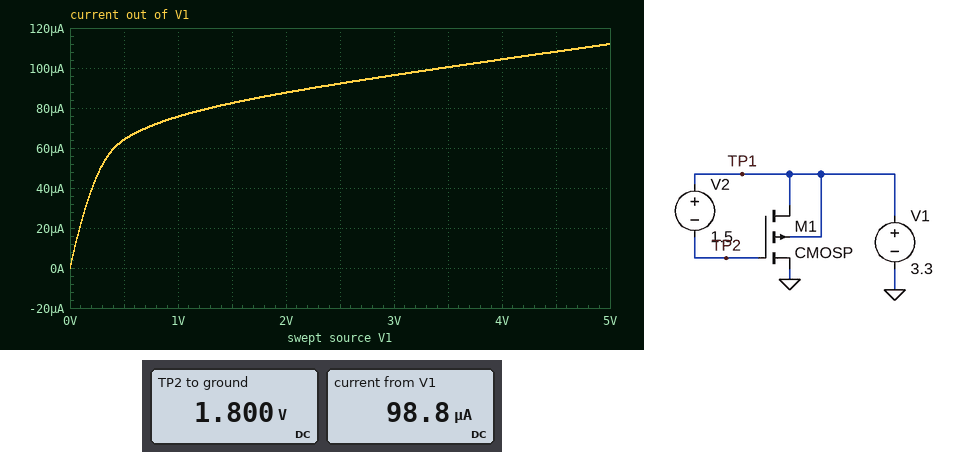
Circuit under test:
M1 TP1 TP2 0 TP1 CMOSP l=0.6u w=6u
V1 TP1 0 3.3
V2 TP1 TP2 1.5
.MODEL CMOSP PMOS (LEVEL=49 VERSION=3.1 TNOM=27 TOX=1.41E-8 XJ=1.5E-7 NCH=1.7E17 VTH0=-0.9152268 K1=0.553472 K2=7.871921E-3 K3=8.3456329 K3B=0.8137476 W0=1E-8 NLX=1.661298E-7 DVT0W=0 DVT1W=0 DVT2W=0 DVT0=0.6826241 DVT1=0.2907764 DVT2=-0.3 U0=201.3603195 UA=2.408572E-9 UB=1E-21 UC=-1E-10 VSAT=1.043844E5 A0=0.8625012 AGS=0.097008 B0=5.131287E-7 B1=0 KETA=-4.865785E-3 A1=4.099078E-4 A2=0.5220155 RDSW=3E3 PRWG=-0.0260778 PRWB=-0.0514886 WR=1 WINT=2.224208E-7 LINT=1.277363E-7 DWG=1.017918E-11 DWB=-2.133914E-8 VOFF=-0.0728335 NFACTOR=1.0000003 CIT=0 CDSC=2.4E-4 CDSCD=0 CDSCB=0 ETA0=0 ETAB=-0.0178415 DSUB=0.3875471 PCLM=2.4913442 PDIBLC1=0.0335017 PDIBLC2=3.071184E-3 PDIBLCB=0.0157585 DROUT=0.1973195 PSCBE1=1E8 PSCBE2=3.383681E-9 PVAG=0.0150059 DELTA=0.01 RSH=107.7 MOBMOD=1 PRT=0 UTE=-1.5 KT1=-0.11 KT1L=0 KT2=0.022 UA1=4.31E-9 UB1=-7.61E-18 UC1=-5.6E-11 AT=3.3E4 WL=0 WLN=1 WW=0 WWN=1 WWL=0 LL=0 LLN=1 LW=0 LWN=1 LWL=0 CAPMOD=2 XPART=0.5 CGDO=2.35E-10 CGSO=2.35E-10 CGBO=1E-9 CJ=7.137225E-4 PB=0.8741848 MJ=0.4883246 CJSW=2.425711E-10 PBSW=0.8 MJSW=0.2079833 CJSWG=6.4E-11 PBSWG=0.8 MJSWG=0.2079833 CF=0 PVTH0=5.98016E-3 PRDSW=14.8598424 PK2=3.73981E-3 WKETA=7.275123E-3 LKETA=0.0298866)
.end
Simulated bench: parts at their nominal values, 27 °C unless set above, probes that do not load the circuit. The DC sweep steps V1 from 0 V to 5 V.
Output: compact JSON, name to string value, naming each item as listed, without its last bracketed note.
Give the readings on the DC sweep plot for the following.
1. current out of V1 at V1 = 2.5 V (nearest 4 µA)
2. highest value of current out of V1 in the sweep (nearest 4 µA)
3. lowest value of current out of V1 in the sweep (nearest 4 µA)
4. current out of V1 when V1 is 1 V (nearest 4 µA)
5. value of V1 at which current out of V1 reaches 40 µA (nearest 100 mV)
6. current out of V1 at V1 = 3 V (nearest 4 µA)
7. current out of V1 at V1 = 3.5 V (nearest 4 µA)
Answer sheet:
{"current out of V1 at V1 = 2.5 V": "92 µA", "highest value of current out of V1 in the sweep": "112 µA", "lowest value of current out of V1 in the sweep": "0 A", "current out of V1 when V1 is 1 V": "76 µA", "value of V1 at which current out of V1 reaches 40 µA": "200 mV", "current out of V1 at V1 = 3 V": "96 µA", "current out of V1 at V1 = 3.5 V": "100 µA"}
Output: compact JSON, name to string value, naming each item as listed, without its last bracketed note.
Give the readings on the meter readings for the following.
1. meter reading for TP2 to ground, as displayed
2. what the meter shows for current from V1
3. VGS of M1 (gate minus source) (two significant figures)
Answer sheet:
{"meter reading for TP2 to ground, as displayed": "1.800 V", "what the meter shows for current from V1": "98.8 µA", "VGS of M1 (gate minus source)": "1.8 V"}
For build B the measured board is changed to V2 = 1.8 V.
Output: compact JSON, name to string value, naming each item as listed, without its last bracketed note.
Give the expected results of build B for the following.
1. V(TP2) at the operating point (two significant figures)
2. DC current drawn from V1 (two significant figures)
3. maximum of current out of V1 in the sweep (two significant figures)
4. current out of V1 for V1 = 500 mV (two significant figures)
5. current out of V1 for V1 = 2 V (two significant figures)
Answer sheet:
{"V(TP2) at the operating point": "1.5 V", "DC current drawn from V1": "190 µA", "maximum of current out of V1 in the sweep": "210 µA", "current out of V1 for V1 = 500 mV": "110 µA", "current out of V1 for V1 = 2 V": "170 µA"}
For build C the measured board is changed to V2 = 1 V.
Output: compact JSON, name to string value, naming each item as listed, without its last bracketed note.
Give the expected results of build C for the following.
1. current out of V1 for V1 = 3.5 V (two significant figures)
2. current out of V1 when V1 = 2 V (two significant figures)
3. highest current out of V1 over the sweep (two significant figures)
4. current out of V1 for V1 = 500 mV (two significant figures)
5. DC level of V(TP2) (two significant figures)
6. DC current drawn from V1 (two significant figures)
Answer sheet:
{"current out of V1 for V1 = 3.5 V": "3.3 µA", "current out of V1 when V1 = 2 V": "2.5 µA", "highest current out of V1 over the sweep": "4.2 µA", "current out of V1 for V1 = 500 mV": "1.7 µA", "DC level of V(TP2)": "2.3 V", "DC current drawn from V1": "3.2 µA"}
